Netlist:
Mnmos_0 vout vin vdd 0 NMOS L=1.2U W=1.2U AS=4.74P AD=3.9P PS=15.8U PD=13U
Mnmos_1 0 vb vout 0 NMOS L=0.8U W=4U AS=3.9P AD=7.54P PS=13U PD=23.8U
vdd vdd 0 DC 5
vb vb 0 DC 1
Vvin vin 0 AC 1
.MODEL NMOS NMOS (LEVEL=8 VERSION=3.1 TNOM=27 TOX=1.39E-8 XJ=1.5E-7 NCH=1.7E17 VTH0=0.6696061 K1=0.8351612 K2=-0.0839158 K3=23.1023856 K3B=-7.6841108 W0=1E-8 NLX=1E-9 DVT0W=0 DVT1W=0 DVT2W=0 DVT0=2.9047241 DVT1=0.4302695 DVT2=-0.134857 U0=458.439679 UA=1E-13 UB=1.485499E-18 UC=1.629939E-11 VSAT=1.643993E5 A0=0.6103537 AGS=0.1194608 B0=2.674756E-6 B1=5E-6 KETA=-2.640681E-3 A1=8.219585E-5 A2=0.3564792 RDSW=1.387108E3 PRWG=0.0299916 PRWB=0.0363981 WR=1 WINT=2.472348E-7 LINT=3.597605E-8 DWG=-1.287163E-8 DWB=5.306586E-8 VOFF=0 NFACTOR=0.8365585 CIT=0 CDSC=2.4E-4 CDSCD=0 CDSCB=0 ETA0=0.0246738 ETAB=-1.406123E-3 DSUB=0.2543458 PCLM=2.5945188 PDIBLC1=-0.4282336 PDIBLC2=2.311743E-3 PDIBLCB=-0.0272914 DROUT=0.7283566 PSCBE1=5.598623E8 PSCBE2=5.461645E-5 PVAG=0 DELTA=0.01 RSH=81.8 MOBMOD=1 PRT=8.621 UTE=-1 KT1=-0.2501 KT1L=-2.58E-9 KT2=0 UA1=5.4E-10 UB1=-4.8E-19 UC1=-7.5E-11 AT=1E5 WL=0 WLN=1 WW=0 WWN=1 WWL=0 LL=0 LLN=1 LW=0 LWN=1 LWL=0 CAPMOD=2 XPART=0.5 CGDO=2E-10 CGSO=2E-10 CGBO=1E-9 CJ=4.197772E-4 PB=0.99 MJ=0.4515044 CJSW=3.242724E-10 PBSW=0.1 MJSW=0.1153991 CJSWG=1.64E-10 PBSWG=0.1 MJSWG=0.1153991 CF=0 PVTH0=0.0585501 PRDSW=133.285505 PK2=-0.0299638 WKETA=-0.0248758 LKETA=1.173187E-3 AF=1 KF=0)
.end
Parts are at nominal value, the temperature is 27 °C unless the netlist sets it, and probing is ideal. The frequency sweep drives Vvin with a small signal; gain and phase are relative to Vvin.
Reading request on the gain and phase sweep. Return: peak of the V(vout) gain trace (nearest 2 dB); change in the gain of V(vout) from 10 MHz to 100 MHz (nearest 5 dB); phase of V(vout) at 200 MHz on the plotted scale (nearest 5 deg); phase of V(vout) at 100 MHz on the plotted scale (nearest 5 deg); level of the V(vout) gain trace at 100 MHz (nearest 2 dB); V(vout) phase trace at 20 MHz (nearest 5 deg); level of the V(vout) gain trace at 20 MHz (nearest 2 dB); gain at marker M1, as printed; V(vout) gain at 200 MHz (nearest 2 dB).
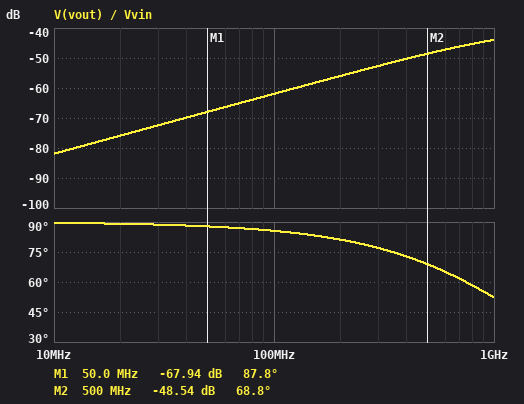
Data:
-44 dB
20 dB
80 deg
85 deg
-62 dB
90 deg
-76 dB
-67.94 dB
-56 dB
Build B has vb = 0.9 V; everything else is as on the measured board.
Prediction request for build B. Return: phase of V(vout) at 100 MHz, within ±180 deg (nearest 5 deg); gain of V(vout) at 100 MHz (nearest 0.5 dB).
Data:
80 deg
-55.5 dB
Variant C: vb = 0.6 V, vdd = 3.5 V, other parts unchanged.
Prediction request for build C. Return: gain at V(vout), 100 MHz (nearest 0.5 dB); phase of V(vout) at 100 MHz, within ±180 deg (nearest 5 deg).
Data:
-38.5 dB
0 deg
